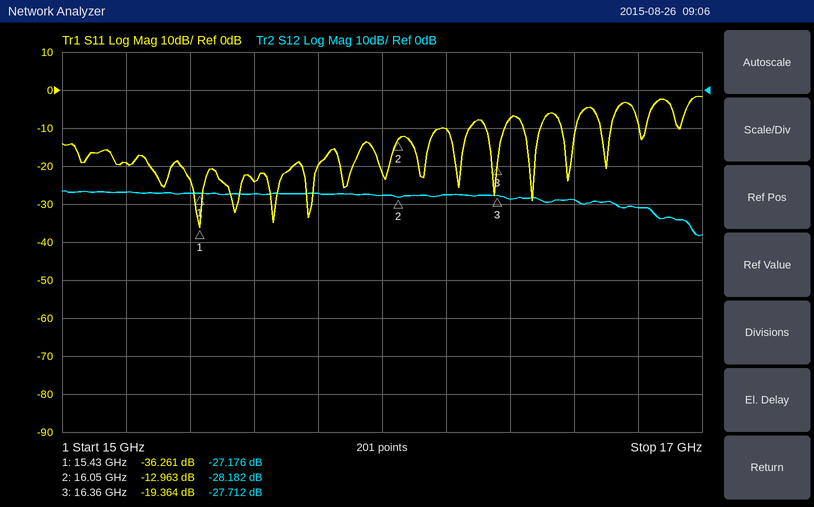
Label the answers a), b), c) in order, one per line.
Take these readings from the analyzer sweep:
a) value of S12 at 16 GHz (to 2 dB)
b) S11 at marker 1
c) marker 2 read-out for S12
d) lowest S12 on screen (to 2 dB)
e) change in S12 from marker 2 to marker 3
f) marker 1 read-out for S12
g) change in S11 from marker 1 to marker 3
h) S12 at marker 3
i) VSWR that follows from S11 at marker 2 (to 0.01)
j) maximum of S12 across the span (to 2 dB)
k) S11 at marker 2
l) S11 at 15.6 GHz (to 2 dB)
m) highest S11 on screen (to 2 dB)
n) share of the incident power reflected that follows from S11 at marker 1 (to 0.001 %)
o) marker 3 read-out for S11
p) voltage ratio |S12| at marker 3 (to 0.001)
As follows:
a) -28 dB
b) -36.261 dB
c) -28.182 dB
d) -38 dB
e) 0.470 dB
f) -27.176 dB
g) 16.897 dB
h) -27.712 dB
i) 1.58
j) -26 dB
k) -12.963 dB
l) -24 dB
m) -2 dB
n) 0.024 %
o) -19.364 dB
p) 0.041
